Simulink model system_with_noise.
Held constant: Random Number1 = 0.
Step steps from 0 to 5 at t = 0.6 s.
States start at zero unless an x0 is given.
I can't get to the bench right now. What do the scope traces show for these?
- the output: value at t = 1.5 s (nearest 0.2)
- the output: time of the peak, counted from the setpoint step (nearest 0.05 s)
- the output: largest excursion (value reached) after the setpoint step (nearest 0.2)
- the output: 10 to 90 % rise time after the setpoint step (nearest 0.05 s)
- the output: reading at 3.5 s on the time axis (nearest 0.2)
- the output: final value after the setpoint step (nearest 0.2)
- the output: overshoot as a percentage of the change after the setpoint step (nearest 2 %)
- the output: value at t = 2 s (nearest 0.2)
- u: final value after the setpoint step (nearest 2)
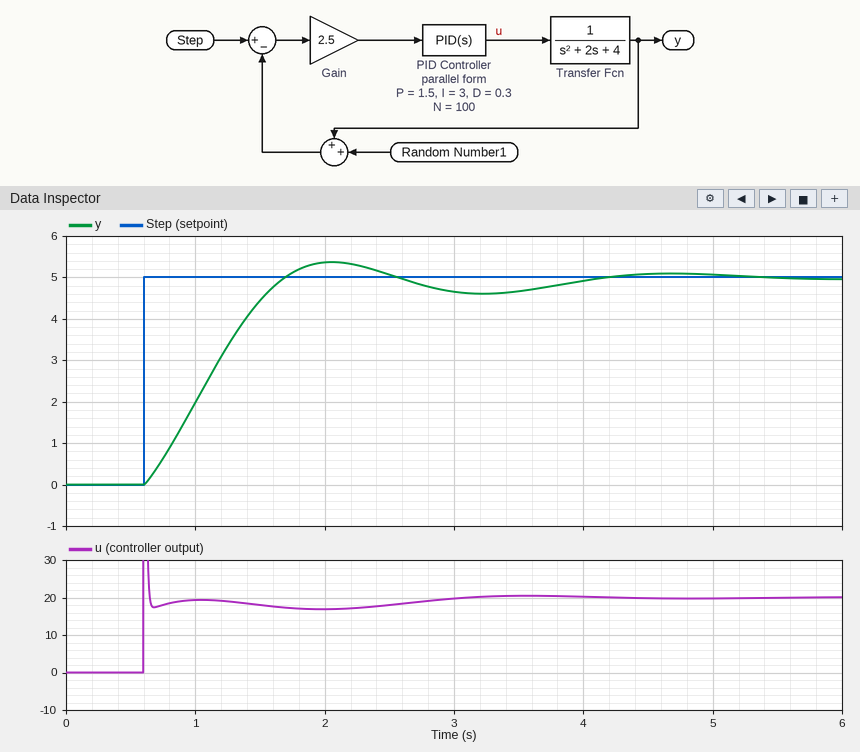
4.4
1.45 s
5.4
0.80 s
4.6
5.0
8 %
5.4
20
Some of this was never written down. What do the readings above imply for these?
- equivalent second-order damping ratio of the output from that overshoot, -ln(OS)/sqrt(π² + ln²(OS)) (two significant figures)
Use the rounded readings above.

0.63
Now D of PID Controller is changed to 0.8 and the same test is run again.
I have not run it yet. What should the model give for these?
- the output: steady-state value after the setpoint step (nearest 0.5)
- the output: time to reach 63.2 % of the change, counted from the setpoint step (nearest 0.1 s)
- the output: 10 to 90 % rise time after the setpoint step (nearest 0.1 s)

5.0
0.5 s
1.2 s
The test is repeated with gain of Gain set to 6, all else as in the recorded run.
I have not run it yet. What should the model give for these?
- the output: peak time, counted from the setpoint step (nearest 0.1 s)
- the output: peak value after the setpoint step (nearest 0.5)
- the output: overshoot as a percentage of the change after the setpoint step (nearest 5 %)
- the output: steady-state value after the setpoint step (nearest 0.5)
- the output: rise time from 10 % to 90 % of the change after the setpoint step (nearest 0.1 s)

0.9 s
6.0
20 %
5.0
0.4 s
